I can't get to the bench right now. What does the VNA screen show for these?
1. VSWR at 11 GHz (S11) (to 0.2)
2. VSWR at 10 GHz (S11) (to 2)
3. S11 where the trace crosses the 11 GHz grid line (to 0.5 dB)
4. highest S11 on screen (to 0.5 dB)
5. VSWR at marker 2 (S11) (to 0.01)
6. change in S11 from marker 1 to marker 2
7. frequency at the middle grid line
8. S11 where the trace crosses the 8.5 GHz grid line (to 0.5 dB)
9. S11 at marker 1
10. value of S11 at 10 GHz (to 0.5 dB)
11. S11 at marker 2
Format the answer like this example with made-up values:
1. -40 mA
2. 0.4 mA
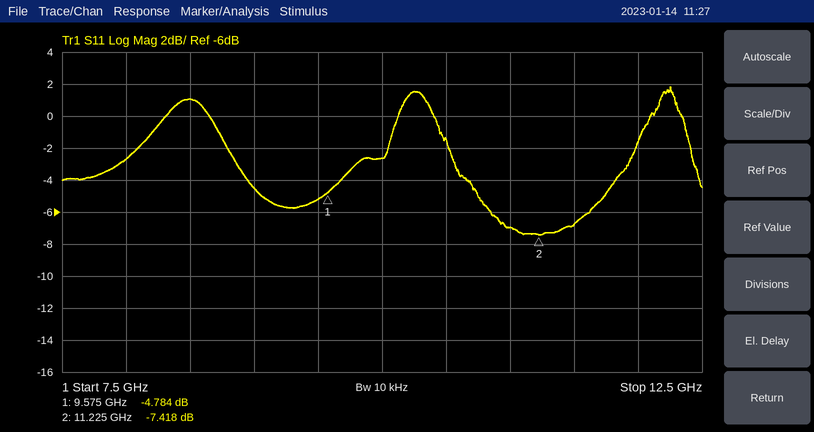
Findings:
1. 2.6
2. 6
3. -7.0 dB
4. 2.0 dB
5. 2.48
6. -2.634 dB
7. 10 GHz
8. 1.0 dB
9. -4.784 dB
10. -2.5 dB
11. -7.418 dB
